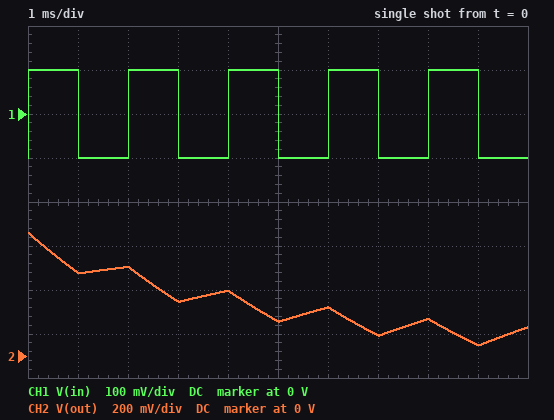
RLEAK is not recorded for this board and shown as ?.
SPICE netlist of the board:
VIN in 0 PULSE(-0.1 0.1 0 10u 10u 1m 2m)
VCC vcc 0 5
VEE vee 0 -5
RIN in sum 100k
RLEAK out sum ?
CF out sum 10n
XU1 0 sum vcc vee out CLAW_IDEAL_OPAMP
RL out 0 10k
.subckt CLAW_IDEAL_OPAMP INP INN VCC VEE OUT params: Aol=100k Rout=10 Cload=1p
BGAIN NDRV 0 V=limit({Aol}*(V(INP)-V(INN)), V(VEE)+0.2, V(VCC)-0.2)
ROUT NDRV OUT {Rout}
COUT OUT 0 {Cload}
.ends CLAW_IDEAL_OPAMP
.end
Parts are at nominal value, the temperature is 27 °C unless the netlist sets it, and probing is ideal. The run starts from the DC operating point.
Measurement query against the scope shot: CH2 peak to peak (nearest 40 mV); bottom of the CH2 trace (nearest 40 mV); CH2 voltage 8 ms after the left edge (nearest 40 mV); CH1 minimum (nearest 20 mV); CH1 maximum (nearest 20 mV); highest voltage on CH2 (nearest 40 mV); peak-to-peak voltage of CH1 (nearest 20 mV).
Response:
520 mV
40 mV
160 mV
-100 mV
100 mV
560 mV
200 mV
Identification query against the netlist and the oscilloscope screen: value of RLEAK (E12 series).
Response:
560 kΩ
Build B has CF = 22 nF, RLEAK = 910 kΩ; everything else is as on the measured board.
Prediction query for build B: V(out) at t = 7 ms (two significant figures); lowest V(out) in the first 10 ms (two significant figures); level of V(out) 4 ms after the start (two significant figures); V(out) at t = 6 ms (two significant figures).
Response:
600 mV
540 mV
750 mV
680 mV
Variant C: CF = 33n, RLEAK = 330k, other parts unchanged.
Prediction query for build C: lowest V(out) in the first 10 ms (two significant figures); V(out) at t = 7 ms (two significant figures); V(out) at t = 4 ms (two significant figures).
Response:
120 mV
150 mV
230 mV
